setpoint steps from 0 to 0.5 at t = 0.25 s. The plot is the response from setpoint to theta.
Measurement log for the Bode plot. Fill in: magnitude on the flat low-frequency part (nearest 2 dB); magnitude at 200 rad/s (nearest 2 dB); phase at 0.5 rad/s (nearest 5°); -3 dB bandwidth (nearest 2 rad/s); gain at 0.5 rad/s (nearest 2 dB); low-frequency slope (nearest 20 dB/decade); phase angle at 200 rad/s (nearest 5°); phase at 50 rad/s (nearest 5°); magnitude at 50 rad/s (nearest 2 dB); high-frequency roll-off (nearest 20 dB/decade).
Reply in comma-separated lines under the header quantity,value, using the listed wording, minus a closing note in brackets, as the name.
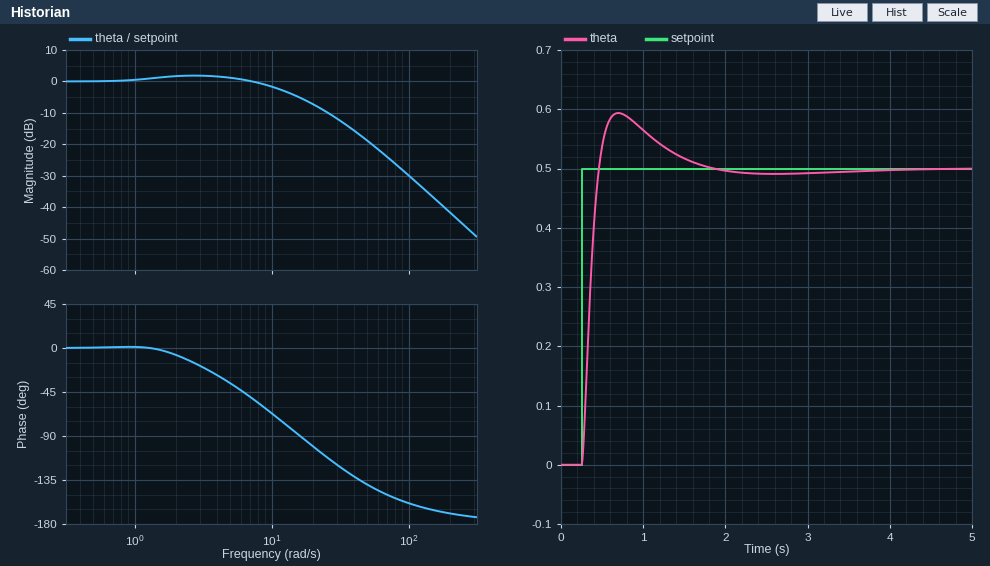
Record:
quantity,value
magnitude on the flat low-frequency part,0 dB
magnitude at 200 rad/s,-42 dB
phase at 0.5 rad/s,0°
-3 dB bandwidth,12 rad/s
gain at 0.5 rad/s,0 dB
low-frequency slope,0 dB/decade
phase angle at 200 rad/s,-170°
phase at 50 rad/s,-140°
magnitude at 50 rad/s,-18 dB
high-frequency roll-off,-40 dB/decade
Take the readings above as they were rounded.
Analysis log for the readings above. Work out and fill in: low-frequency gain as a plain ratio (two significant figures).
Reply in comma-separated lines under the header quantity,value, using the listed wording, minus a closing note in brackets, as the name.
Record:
quantity,value
low-frequency gain as a plain ratio,1.0
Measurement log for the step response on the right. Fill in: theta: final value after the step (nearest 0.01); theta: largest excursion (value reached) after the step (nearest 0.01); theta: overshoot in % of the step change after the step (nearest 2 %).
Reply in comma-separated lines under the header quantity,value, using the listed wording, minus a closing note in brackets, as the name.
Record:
quantity,value
theta: final value after the step,0.50
theta: largest excursion (value reached) after the step,0.59
theta: overshoot in % of the step change after the step,18 %
